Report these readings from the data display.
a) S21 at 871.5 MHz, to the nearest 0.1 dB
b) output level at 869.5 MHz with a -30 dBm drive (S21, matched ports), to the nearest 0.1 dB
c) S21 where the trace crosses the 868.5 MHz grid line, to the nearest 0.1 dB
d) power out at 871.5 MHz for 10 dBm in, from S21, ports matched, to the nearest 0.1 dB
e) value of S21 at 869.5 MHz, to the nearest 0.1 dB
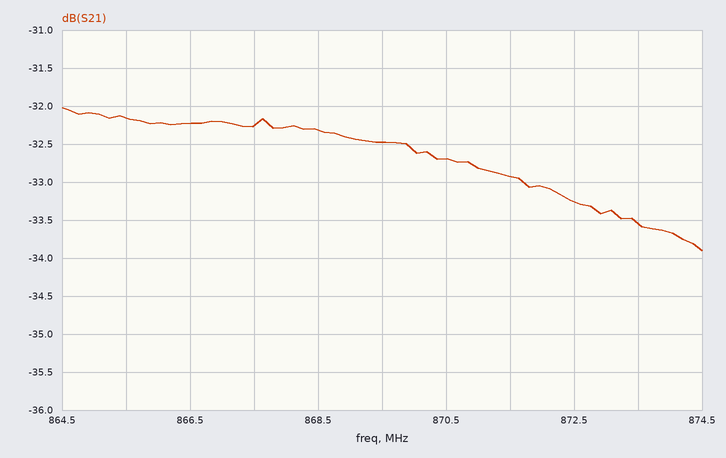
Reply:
-32.9 dB
-62.5 dBm
-32.3 dB
-22.9 dBm
-32.5 dB
